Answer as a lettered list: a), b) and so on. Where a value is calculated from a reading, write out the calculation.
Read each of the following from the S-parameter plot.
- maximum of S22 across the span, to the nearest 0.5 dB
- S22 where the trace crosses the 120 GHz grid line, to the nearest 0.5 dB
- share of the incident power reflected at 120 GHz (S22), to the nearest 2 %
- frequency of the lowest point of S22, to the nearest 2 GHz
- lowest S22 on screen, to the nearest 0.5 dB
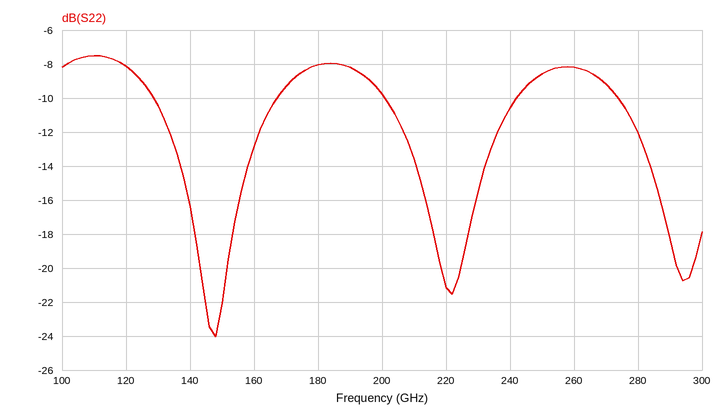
a) -7.5 dB
b) -8.0 dB
c) 10^(-8/10) ≈ 16 %
d) 148 GHz
e) -24.0 dB
